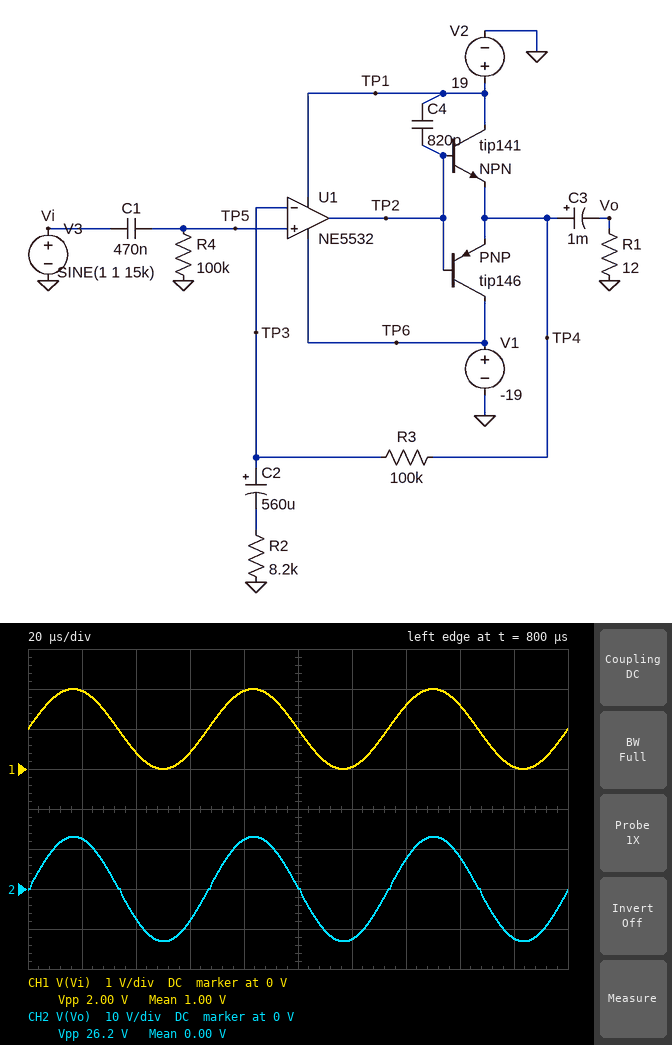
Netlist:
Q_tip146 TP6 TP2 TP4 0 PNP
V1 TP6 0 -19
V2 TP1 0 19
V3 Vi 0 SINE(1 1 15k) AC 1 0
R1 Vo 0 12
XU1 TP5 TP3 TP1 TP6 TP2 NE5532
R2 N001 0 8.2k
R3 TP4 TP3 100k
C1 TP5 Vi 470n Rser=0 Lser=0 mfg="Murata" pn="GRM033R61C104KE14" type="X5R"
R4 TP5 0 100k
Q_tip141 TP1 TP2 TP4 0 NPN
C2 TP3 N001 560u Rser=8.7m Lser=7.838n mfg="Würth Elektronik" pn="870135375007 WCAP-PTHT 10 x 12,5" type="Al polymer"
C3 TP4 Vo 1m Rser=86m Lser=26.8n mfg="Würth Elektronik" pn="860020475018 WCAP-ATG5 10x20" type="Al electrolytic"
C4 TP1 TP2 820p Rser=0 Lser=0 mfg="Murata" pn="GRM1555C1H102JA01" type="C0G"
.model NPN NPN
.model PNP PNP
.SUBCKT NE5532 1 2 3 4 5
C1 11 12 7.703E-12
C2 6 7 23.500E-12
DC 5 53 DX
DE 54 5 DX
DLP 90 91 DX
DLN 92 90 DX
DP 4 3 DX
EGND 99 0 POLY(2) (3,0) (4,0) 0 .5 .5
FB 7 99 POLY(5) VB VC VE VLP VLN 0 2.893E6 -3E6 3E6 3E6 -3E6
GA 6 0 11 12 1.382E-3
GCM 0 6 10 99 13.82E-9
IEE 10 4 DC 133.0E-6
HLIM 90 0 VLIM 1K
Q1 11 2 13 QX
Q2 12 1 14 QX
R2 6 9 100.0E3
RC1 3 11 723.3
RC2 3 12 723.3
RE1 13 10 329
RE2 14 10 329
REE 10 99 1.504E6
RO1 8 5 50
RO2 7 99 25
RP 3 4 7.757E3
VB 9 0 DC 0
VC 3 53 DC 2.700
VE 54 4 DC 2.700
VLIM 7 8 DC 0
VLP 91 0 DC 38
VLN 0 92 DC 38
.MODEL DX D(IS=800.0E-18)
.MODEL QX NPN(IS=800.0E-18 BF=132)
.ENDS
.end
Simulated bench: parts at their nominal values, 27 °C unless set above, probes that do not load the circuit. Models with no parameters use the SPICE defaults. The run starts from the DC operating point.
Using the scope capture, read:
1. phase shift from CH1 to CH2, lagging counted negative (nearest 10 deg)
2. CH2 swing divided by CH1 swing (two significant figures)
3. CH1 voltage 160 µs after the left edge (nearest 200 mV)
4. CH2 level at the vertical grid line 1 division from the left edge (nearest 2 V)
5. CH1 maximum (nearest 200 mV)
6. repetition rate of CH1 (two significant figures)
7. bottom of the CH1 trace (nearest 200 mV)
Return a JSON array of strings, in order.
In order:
["0 deg", "13", "1.6 V", "12 V", "2.0 V", "15 kHz", "0 V"]
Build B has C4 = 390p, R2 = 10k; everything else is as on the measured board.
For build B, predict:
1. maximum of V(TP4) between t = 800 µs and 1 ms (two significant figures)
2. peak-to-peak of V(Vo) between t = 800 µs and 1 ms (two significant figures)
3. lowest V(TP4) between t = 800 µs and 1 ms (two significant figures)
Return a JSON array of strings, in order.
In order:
["11 V", "22 V", "-11 V"]
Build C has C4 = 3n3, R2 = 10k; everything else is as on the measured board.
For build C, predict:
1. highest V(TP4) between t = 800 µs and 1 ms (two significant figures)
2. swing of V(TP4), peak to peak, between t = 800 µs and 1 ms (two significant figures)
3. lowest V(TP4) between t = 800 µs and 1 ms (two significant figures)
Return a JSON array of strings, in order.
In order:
["11 V", "22 V", "-11 V"]
